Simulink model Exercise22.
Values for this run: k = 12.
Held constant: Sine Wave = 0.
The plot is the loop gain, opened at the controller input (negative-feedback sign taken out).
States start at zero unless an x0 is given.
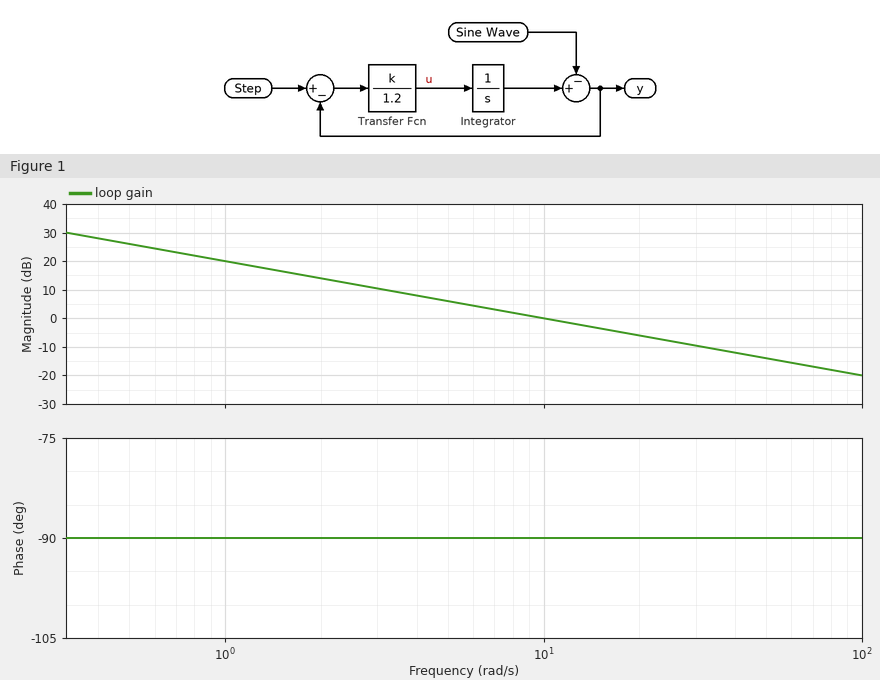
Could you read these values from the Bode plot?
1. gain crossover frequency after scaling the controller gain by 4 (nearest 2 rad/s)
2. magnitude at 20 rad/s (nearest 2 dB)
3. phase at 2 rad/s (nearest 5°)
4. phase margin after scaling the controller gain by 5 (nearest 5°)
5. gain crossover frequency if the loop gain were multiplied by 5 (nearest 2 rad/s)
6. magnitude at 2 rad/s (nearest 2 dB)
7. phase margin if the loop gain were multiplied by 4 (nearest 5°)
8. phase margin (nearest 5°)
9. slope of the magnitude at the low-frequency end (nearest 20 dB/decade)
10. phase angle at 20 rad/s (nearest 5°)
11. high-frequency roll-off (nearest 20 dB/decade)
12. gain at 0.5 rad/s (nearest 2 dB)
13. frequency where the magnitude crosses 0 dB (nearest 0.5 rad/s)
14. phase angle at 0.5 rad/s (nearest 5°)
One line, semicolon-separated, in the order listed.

40 rad/s; -6 dB; -90°; 90°; 50 rad/s; 14 dB; 90°; 90°; -20 dB/decade; -90°; -20 dB/decade; 26 dB; 10.0 rad/s; -90°
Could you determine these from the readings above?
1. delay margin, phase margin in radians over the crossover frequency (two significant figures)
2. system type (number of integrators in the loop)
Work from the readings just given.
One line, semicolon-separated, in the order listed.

0.16 s; 1
